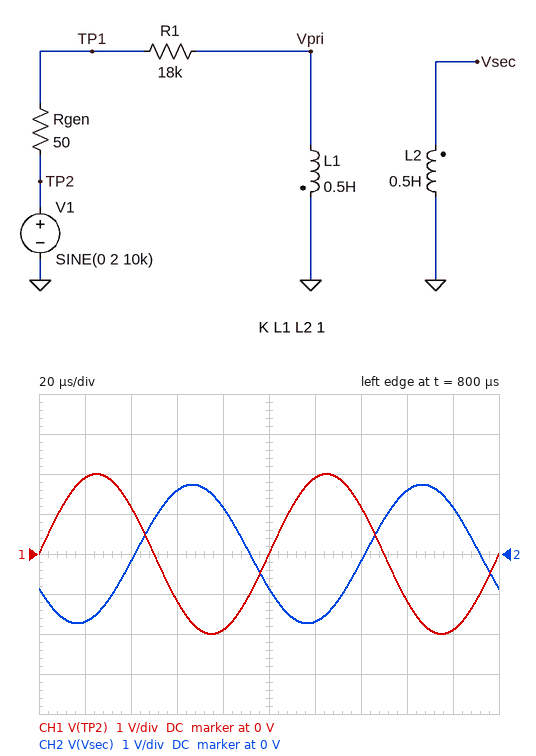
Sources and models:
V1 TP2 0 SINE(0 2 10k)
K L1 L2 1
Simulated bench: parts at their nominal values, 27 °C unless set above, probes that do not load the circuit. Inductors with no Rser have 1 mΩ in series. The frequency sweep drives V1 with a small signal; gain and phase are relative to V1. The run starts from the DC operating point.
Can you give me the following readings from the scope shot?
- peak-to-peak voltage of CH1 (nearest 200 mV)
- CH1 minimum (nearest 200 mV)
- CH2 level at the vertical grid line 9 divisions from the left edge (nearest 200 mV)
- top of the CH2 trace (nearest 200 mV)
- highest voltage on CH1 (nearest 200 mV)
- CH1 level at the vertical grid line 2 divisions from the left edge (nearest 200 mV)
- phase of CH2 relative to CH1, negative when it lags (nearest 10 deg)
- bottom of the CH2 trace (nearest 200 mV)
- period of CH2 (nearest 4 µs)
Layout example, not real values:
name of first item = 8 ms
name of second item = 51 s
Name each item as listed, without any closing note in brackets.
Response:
peak-to-peak voltage of CH1 = 4.0 V
CH1 minimum = -2.0 V
CH2 level at the vertical grid line 9 divisions from the left edge = 1.2 V
top of the CH2 trace = 1.8 V
highest voltage on CH1 = 2.0 V
CH1 level at the vertical grid line 2 divisions from the left edge = 1.2 V
phase of CH2 relative to CH1, negative when it lags = -150 deg
bottom of the CH2 trace = -1.8 V
period of CH2 = 100 µs
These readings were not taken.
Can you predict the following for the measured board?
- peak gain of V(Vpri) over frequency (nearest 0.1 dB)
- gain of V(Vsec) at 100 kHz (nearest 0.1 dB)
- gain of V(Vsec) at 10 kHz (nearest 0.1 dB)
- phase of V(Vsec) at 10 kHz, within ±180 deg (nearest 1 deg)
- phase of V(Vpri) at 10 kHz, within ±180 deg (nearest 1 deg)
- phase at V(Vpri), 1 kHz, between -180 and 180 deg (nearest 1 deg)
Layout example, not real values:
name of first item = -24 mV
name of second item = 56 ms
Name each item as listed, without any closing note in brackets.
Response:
peak gain of V(Vpri) over frequency = 0 dB
gain of V(Vsec) at 100 kHz = 0 dB
gain of V(Vsec) at 10 kHz = -1.2 dB
phase of V(Vsec) at 10 kHz, within ±180 deg = -150 deg
phase of V(Vpri) at 10 kHz, within ±180 deg = 30 deg
phase at V(Vpri), 1 kHz, between -180 and 180 deg = 80 deg
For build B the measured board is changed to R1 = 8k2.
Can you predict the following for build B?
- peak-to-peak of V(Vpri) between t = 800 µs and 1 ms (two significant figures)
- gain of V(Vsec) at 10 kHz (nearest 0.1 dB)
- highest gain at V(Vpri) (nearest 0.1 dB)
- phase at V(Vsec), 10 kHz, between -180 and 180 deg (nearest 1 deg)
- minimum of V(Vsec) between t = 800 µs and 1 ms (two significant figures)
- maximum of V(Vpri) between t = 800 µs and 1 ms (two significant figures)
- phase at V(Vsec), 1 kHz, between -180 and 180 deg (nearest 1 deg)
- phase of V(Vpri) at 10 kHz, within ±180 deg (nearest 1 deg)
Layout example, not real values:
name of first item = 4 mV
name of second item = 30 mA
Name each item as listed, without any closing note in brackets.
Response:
peak-to-peak of V(Vpri) between t = 800 µs and 1 ms = 3.9 V
gain of V(Vsec) at 10 kHz = -0.3 dB
highest gain at V(Vpri) = 0 dB
phase at V(Vsec), 10 kHz, between -180 and 180 deg = -165 deg
minimum of V(Vsec) between t = 800 µs and 1 ms = -1.9 V
maximum of V(Vpri) between t = 800 µs and 1 ms = 1.9 V
phase at V(Vsec), 1 kHz, between -180 and 180 deg = -111 deg
phase of V(Vpri) at 10 kHz, within ±180 deg = 15 deg
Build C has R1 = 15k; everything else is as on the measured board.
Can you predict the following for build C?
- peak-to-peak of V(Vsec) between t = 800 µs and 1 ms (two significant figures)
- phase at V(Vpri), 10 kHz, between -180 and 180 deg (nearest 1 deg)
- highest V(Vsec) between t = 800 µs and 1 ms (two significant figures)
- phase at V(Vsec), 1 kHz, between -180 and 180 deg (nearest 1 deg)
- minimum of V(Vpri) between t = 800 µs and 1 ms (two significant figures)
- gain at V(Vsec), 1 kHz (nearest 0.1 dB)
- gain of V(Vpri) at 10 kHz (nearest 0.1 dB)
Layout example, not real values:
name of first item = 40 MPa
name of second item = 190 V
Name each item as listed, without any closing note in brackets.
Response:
peak-to-peak of V(Vsec) between t = 800 µs and 1 ms = 3.6 V
phase at V(Vpri), 10 kHz, between -180 and 180 deg = 26 deg
highest V(Vsec) between t = 800 µs and 1 ms = 1.8 V
phase at V(Vsec), 1 kHz, between -180 and 180 deg = -102 deg
minimum of V(Vpri) between t = 800 µs and 1 ms = -1.8 V
gain at V(Vsec), 1 kHz = -13.8 dB
gain of V(Vpri) at 10 kHz = -0.9 dB
